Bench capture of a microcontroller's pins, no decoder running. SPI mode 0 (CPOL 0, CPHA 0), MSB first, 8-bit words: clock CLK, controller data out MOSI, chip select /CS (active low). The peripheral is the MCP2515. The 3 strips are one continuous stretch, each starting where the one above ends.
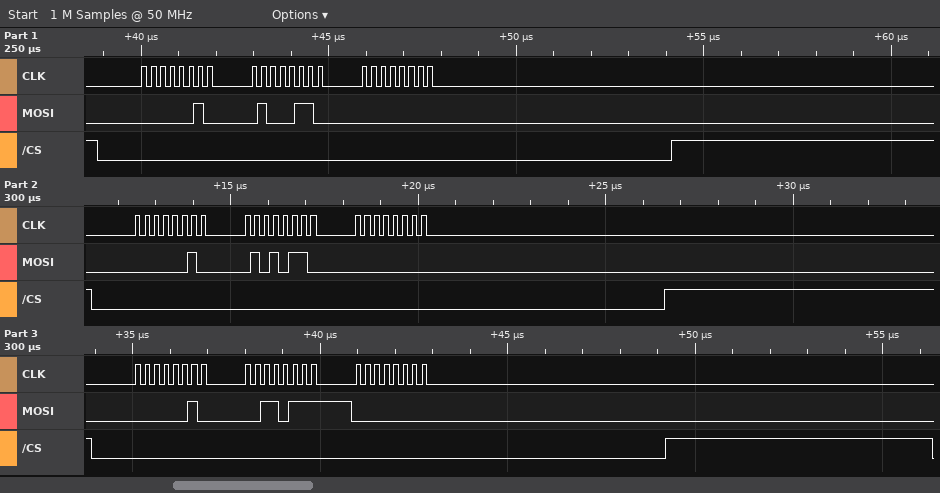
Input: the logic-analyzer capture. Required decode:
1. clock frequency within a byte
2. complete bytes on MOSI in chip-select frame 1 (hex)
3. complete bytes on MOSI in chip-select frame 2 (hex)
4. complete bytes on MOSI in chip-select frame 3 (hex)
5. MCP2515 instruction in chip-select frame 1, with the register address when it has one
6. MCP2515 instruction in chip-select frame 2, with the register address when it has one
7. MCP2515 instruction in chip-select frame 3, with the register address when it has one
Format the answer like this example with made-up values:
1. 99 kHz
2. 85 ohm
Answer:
1. 4 MHz
2. 0x02 0x46 0x00
3. 0x02 0x56 0x00
4. 0x02 0x37 0x00
5. WRITE 0x46
6. WRITE 0x56
7. WRITE 0x37
